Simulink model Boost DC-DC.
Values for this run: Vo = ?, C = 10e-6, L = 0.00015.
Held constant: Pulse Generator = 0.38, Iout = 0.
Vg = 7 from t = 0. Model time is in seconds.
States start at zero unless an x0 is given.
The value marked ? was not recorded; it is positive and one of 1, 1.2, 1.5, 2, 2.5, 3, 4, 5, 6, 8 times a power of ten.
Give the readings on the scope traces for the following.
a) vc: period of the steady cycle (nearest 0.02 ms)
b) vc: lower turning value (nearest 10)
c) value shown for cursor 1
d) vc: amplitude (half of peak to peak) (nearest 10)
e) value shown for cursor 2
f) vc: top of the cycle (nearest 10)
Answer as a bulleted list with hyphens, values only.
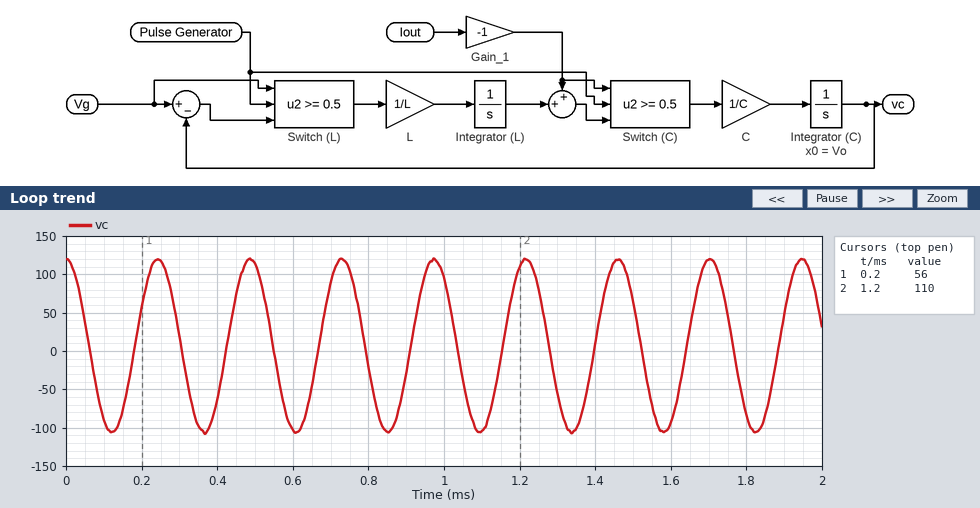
- 0.24 ms
- -110
- 56
- 110
- 110
- 120
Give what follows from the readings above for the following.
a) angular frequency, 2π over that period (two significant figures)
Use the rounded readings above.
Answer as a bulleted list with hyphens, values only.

- 26 rad/ms
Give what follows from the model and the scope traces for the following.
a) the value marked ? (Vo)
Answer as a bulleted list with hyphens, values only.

- 120
